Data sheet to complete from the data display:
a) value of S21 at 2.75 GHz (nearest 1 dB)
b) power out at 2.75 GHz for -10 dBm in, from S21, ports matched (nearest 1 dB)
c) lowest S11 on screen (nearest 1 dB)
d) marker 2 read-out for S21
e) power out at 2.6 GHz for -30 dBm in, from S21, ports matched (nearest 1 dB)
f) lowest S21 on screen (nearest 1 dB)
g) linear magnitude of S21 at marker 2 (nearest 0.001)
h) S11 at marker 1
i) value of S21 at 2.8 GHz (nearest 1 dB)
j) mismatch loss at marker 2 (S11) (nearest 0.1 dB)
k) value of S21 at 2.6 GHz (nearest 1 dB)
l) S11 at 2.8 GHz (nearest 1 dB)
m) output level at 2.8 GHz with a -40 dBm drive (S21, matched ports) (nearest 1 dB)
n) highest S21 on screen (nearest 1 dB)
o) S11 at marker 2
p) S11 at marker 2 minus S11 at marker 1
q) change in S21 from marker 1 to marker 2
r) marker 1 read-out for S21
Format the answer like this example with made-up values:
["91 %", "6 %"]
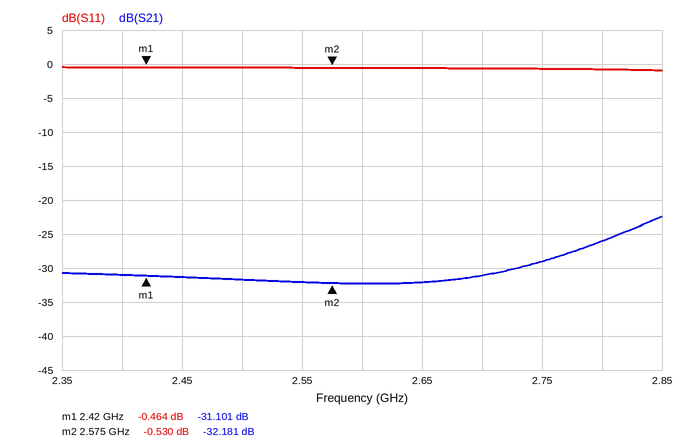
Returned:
["-29 dB", "-39 dBm", "-1 dB", "-32.181 dB", "-62 dBm", "-32 dB", "0.025", "-0.464 dB", "-26 dB", "9.4 dB", "-32 dB", "-1 dB", "-66 dBm", "-22 dB", "-0.530 dB", "-0.066 dB", "-1.080 dB", "-31.101 dB"]
